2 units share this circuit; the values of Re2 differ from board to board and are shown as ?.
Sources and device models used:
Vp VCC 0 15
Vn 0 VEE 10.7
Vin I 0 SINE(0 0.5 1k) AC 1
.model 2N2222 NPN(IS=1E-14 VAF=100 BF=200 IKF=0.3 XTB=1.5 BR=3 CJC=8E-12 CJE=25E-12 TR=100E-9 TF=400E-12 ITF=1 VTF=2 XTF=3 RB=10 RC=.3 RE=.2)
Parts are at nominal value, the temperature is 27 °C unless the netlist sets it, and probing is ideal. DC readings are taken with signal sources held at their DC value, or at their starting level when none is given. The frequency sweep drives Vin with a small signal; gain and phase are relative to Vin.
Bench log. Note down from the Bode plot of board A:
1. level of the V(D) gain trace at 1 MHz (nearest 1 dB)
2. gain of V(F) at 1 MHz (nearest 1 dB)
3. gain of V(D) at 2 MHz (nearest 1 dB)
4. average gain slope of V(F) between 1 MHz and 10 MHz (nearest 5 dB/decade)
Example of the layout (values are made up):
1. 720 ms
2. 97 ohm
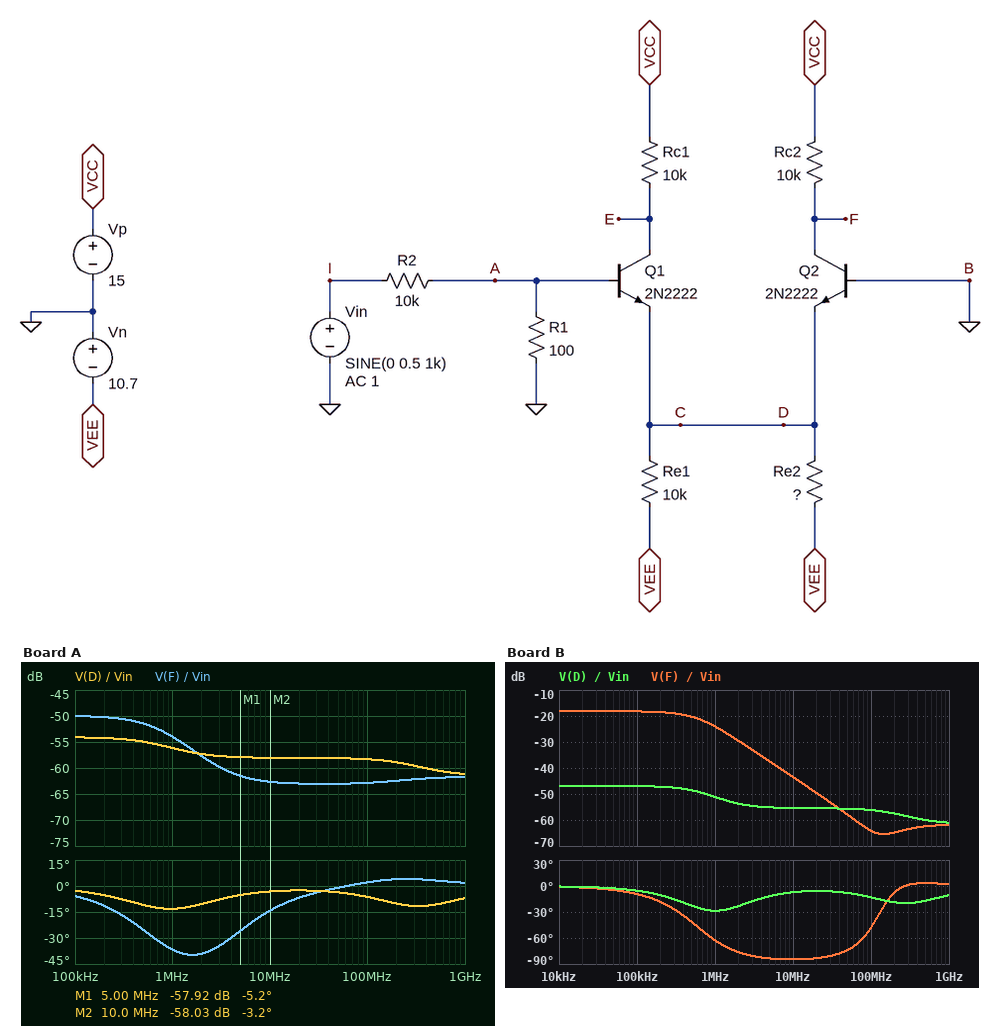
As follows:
1. -56 dB
2. -54 dB
3. -57 dB
4. -10 dB/decade
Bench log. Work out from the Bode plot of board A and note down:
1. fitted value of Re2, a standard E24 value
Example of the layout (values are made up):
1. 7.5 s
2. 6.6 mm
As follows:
1. 3.6 kΩ
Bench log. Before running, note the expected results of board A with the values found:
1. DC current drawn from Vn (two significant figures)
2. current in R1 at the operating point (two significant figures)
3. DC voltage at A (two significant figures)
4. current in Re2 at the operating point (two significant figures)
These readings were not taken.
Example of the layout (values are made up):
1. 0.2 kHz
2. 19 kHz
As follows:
1. 3.8 mA
2. 160 µA
3. -16 mV
4. 2.8 mA
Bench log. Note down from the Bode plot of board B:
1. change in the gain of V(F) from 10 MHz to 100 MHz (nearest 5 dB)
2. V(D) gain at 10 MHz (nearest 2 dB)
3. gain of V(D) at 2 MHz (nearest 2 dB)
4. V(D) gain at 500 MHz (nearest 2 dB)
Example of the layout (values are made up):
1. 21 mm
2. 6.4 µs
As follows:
1. -20 dB
2. -56 dB
3. -54 dB
4. -60 dB
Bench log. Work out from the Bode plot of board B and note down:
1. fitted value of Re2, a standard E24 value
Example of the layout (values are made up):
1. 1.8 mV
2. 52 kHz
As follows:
1. 4.7 kΩ
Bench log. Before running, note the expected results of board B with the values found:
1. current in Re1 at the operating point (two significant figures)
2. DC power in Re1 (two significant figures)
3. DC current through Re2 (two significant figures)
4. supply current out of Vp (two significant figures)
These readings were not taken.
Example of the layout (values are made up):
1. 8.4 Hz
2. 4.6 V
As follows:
1. 1.0 mA
2. 10 mW
3. 2.1 mA
4. 3.1 mA
